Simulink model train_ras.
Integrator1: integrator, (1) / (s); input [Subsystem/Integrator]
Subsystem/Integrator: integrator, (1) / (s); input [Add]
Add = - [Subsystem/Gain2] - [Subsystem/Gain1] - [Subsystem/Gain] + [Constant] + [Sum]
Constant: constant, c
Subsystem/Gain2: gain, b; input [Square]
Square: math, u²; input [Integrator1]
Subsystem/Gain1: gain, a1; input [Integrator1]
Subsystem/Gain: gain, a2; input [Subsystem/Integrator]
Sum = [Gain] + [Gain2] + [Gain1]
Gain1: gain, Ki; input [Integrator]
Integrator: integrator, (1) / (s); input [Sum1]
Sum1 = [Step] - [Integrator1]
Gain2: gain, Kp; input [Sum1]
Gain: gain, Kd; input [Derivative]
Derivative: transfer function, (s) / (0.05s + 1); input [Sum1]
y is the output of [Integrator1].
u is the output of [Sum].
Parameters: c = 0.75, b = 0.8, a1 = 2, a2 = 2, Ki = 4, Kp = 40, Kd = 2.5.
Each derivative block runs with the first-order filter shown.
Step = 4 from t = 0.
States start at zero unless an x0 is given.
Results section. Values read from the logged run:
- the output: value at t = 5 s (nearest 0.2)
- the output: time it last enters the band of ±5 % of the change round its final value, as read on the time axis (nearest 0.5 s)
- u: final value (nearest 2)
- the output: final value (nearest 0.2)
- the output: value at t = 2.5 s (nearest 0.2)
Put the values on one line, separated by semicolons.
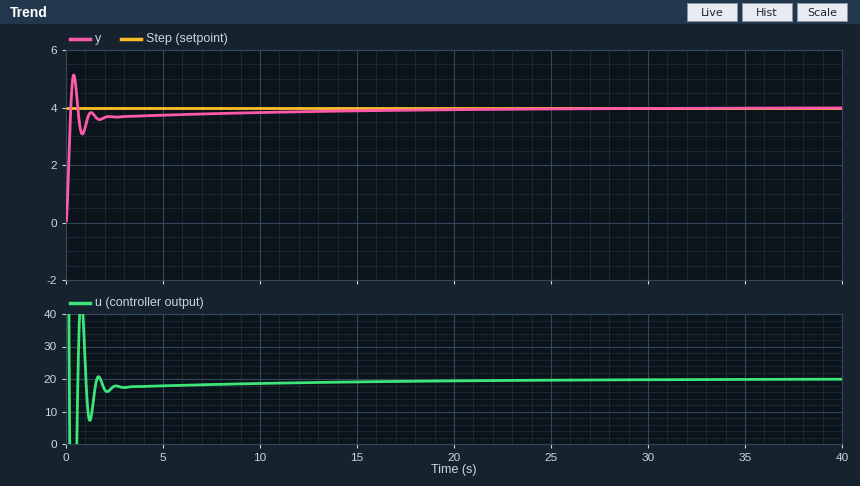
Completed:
3.8; 8.5 s; 20; 4.0; 3.6
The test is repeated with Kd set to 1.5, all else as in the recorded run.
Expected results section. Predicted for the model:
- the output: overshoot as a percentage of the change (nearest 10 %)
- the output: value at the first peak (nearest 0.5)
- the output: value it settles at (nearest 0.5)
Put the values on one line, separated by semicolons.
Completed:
30 %; 5.5; 4.0
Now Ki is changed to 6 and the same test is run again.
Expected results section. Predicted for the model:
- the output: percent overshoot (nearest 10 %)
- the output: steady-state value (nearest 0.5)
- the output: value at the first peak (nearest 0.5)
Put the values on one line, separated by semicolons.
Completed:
30 %; 4.0; 5.0
